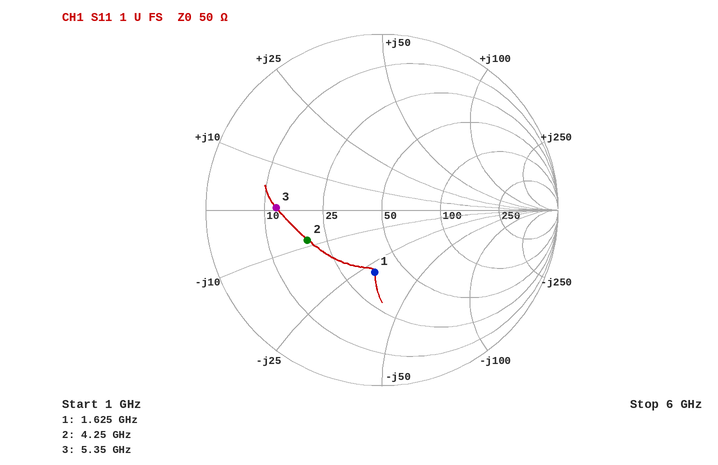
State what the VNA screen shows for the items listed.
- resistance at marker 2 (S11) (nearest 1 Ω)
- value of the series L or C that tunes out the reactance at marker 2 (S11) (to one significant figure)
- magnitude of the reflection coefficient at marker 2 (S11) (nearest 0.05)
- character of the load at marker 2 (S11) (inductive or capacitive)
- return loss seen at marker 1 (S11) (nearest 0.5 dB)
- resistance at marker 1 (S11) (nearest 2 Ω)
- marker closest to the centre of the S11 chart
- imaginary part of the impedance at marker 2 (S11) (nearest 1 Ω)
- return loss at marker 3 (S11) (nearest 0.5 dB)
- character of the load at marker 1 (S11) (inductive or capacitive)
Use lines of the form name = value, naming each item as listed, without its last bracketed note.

resistance at marker 2 (S11) = 19 Ω
value of the series L or C that tunes out the reactance at marker 2 (S11) = 300 pH
magnitude of the reflection coefficient at marker 2 (S11) = 0.45
character of the load at marker 2 (S11) = capacitive
return loss seen at marker 1 (S11) = 9.0 dB
resistance at marker 1 (S11) = 36 Ω
marker closest to the centre of the S11 chart = marker 1
imaginary part of the impedance at marker 2 (S11) = -8 Ω
return loss at marker 3 (S11) = 4.5 dB
character of the load at marker 1 (S11) = capacitive
